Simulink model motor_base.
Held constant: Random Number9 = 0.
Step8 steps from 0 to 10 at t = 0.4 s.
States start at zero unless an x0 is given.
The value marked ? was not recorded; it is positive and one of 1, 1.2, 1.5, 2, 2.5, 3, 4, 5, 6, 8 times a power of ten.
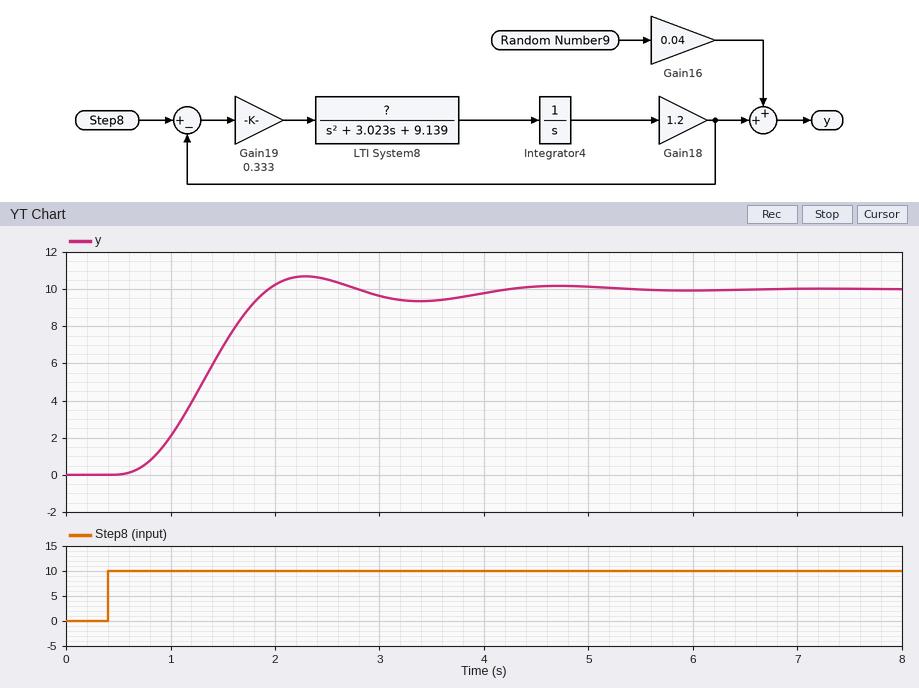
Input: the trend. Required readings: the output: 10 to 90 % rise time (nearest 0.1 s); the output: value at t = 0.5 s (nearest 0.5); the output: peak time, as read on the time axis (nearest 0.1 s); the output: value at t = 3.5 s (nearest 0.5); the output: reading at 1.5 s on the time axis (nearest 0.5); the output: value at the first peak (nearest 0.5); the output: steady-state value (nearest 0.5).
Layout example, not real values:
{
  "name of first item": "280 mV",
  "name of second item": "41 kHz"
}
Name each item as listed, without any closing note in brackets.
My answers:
{
  "the output: 10 to 90 % rise time": "0.9 s",
  "the output: value at t = 0.5 s": "0.0",
  "the output: peak time, as read on the time axis": "2.3 s",
  "the output: value at t = 3.5 s": "9.5",
  "the output: reading at 1.5 s on the time axis": "7.0",
  "the output: value at the first peak": "10.5",
  "the output: steady-state value": "10.0"
}
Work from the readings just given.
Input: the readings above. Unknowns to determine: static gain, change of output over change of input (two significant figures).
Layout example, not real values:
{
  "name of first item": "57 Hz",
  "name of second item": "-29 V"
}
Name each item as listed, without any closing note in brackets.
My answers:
{
  "static gain, change of output over change of input": "1.0"
}
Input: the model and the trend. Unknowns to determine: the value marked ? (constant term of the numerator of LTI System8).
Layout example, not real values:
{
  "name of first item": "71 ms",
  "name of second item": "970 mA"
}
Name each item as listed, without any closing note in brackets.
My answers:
{
  "the value marked ?": "25"
}
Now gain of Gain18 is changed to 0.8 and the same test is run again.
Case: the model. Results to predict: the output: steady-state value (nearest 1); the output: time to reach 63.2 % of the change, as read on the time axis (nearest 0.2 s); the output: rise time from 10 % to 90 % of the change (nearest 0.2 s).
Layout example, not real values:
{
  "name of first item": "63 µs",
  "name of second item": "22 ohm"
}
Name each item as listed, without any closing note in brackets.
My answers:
{
  "the output: steady-state value": "10",
  "the output: time to reach 63.2 % of the change, as read on the time axis": "1.8 s",
  "the output: rise time from 10 % to 90 % of the change": "2.0 s"
}
